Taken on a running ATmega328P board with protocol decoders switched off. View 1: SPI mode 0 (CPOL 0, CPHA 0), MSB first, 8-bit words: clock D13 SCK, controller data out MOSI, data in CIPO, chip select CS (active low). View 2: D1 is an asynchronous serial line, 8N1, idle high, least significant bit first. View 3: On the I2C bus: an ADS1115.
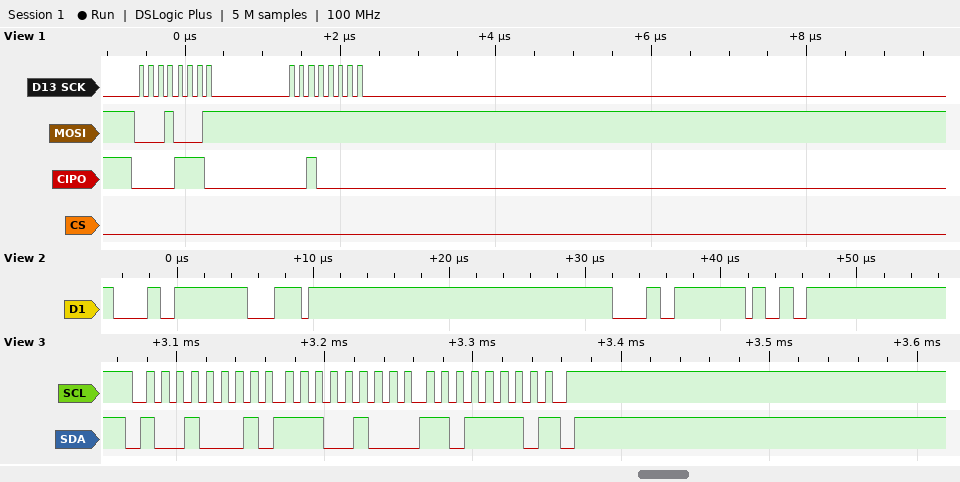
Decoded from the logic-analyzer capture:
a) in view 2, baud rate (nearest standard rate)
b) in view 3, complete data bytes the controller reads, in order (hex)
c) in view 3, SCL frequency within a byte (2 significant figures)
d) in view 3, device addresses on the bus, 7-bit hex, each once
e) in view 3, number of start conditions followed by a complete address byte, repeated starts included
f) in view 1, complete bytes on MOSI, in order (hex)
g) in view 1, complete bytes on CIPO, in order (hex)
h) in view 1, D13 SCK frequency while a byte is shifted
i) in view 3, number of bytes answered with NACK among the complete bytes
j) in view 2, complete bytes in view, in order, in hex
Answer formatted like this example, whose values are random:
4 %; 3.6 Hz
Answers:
2000000 baud; E4 DE; 100 kHz; 0x48; 1; 0x11 0xFF; 0x0E 0x20; 8 MHz; 1; 30 78 30 33
